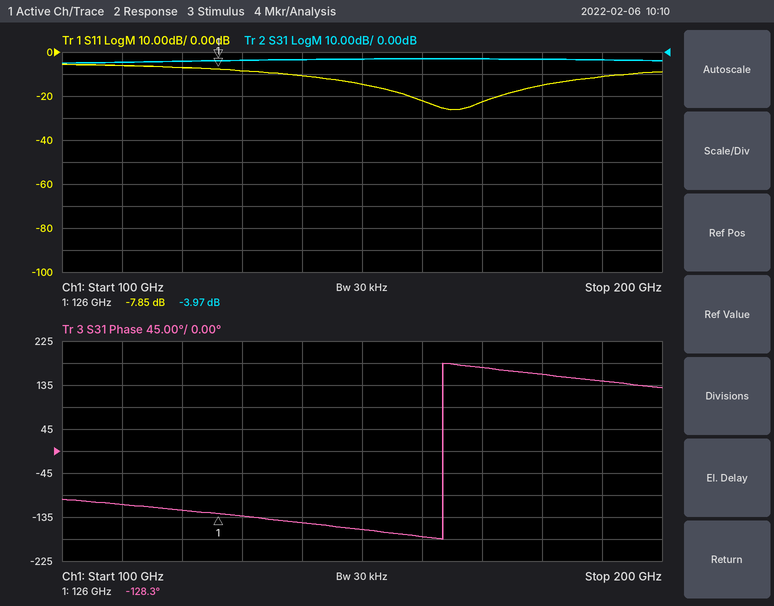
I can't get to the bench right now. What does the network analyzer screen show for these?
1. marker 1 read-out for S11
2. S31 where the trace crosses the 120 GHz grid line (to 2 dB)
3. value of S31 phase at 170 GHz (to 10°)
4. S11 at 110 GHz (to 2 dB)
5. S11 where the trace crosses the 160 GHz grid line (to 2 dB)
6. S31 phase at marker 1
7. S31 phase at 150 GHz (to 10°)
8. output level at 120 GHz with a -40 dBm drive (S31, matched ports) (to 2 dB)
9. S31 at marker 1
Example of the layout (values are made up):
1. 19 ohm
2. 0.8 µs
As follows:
1. -7.85 dB
2. -4 dB
3. 170°
4. -6 dB
5. -22 dB
6. -128.3°
7. -160°
8. -44 dBm
9. -3.97 dB
